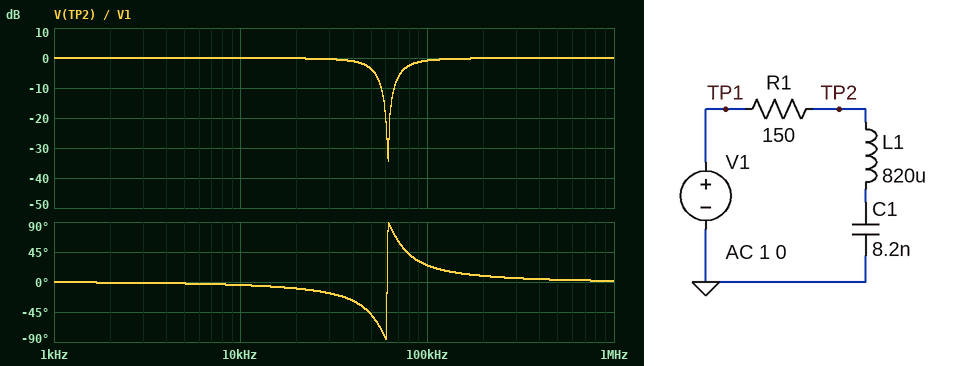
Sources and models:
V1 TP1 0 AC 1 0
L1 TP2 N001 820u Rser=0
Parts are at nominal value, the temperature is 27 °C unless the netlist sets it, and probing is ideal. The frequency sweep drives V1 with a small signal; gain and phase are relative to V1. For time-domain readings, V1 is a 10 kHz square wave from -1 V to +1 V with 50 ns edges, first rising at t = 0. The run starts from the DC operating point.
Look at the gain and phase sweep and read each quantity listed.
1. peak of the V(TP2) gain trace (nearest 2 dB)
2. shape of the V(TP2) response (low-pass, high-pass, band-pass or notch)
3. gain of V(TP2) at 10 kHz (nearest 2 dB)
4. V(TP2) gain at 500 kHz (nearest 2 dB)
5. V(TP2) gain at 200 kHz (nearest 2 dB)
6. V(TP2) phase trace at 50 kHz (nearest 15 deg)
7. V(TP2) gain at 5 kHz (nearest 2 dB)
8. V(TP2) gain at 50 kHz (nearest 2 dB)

0 dB
notch
0 dB
0 dB
0 dB
-45 deg
0 dB
-4 dB
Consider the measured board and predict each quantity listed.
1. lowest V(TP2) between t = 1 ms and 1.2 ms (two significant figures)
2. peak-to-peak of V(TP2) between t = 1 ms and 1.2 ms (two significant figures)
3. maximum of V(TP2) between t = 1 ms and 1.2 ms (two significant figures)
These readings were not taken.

-1.3 V
2.6 V
1.3 V
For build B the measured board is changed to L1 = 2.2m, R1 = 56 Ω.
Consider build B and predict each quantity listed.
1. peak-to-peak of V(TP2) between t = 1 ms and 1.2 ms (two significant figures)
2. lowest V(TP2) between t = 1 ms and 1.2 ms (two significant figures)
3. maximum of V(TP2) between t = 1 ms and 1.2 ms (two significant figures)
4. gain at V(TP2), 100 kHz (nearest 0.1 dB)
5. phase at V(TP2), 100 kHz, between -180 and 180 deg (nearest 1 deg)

2.2 V
-1.1 V
1.1 V
0 dB
3 deg
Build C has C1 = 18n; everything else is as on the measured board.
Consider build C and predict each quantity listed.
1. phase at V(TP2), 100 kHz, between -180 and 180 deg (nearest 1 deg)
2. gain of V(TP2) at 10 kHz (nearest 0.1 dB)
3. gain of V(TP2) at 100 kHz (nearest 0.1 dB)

19 deg
-0.1 dB
-0.5 dB
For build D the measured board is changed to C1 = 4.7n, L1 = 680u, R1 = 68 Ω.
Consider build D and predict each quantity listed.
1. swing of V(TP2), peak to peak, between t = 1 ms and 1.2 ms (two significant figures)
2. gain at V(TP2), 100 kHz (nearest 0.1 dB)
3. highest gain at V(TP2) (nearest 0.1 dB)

2.5 V
-2.0 dB
0 dB
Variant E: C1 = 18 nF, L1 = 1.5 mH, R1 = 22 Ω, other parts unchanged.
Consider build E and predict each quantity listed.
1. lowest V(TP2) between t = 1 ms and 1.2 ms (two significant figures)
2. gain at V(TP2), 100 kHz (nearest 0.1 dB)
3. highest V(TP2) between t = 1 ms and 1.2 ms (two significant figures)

-1.4 V
0 dB
1.4 V
